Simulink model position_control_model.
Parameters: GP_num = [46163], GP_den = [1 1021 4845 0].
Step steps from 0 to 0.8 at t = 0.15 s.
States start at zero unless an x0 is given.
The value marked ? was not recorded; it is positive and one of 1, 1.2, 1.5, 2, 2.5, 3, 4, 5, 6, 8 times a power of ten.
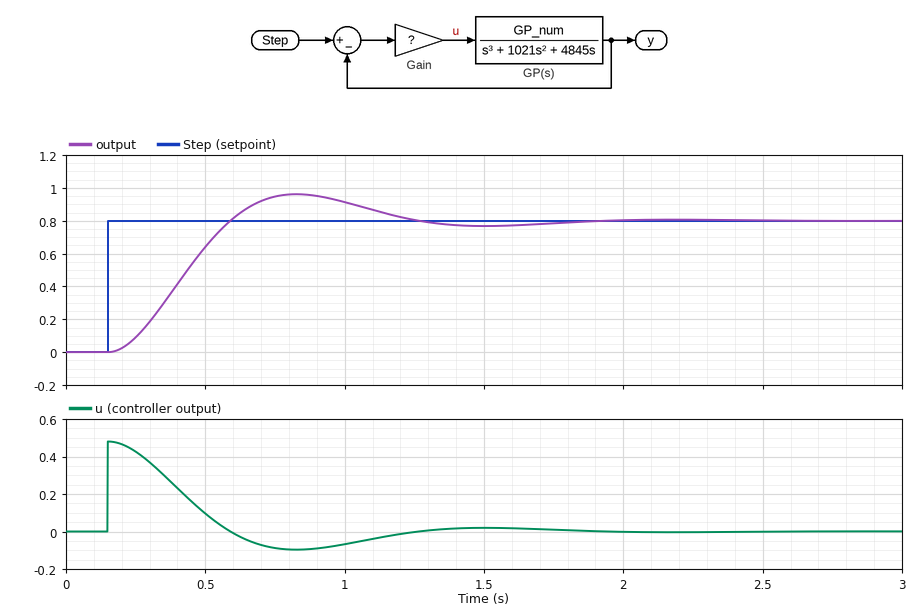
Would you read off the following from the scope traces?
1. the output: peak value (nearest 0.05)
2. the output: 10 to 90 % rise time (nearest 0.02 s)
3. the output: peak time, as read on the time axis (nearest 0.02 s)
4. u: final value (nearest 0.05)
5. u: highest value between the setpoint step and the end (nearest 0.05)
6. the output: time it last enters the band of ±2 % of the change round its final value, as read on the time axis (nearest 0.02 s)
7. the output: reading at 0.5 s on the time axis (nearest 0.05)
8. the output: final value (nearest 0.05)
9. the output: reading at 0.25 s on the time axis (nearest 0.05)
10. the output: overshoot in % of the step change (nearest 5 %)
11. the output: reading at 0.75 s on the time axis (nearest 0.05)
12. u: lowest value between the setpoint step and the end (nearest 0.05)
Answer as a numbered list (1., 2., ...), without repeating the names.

1. 0.95
2. 0.30 s
3. 0.82 s
4. 0.00
5. 0.50
6. 1.74 s
7. 0.65
8. 0.80
9. 0.10
10. 20 %
11. 0.95
12. -0.10
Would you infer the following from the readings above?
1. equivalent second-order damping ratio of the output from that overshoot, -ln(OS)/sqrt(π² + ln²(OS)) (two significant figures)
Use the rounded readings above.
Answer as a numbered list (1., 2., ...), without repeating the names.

1. 0.46
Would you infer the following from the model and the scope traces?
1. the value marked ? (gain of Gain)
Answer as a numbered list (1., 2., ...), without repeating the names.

1. 0.6
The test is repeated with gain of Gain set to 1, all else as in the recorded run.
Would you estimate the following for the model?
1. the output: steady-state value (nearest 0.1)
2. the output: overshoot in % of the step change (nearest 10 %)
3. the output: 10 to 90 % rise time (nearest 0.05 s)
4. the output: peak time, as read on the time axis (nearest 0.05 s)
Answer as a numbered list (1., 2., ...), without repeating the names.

1. 0.8
2. 30 %
3. 0.20 s
4. 0.65 s
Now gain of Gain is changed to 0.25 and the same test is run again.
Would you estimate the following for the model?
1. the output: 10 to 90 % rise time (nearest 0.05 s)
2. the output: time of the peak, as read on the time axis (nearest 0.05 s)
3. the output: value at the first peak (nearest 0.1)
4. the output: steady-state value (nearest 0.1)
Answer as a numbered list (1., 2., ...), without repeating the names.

1. 0.65 s
2. 1.45 s
3. 0.8
4. 0.8
